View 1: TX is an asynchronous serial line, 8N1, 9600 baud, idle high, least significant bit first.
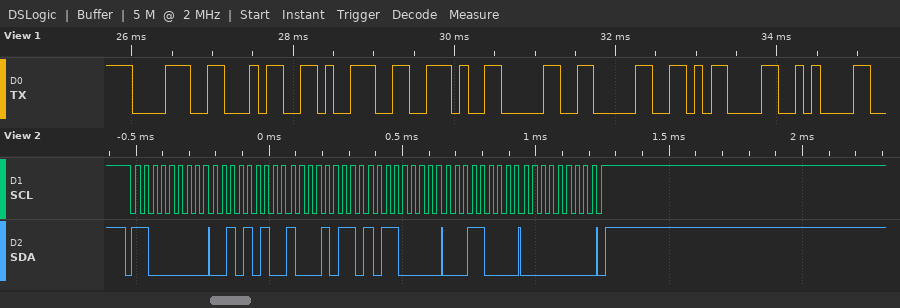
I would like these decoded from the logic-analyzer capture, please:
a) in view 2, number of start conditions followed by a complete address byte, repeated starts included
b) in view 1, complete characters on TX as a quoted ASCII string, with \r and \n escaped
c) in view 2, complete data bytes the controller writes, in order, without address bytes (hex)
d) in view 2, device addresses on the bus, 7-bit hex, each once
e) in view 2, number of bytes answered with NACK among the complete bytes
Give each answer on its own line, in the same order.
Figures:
1
"849.00\r\n"
2A 8B B0 18 00
0x60
0
